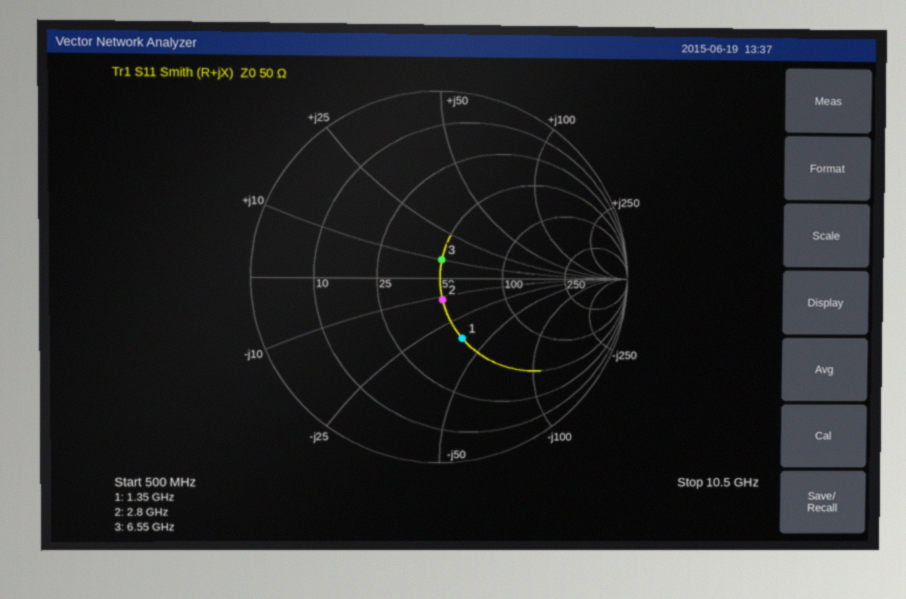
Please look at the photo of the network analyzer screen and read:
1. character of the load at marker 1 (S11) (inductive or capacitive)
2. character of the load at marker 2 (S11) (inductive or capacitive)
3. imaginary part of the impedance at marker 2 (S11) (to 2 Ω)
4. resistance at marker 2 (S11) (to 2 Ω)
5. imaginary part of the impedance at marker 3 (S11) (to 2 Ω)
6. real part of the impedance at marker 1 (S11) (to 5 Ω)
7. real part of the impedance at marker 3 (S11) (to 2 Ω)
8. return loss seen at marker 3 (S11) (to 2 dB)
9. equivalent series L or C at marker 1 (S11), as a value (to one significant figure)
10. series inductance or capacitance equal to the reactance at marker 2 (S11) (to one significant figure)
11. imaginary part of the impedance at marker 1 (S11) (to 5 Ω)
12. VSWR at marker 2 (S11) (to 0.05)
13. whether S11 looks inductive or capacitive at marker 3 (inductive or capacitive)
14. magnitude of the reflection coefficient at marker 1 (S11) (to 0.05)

capacitive
capacitive
-12 Ω
50 Ω
+10 Ω
50 Ω
50 Ω
20 dB
3 pF
5 pF
-35 Ω
1.25
inductive
0.35
